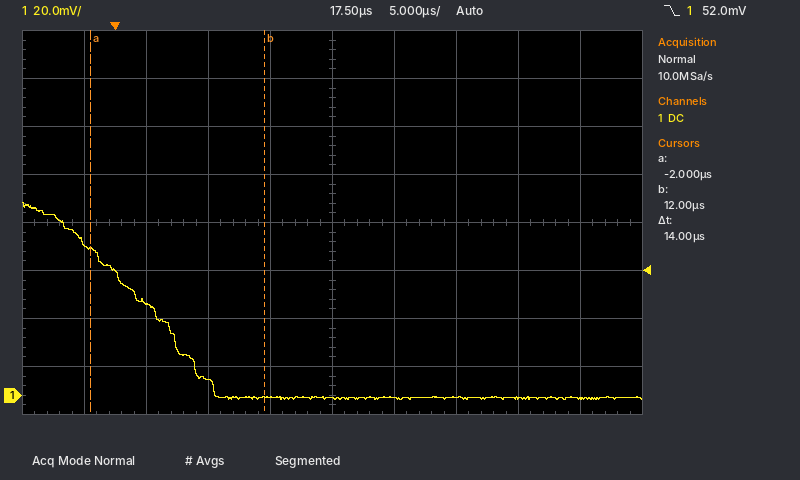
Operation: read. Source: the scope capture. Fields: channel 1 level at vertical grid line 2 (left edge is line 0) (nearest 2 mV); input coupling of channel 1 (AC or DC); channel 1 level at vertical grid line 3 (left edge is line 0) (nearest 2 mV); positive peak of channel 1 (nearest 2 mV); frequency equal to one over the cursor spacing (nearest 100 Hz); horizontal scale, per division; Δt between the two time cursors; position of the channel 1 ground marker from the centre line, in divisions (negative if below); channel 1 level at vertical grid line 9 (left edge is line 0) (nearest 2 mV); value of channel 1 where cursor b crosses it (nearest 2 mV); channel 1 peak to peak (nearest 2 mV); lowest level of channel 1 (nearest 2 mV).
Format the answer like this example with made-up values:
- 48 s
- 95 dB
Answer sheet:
- 38 mV
- DC
- 6 mV
- 80 mV
- 71.4 kHz
- 5 µs
- 14 µs
- -3.6 div
- -2 mV
- 0 mV
- 82 mV
- -2 mV
